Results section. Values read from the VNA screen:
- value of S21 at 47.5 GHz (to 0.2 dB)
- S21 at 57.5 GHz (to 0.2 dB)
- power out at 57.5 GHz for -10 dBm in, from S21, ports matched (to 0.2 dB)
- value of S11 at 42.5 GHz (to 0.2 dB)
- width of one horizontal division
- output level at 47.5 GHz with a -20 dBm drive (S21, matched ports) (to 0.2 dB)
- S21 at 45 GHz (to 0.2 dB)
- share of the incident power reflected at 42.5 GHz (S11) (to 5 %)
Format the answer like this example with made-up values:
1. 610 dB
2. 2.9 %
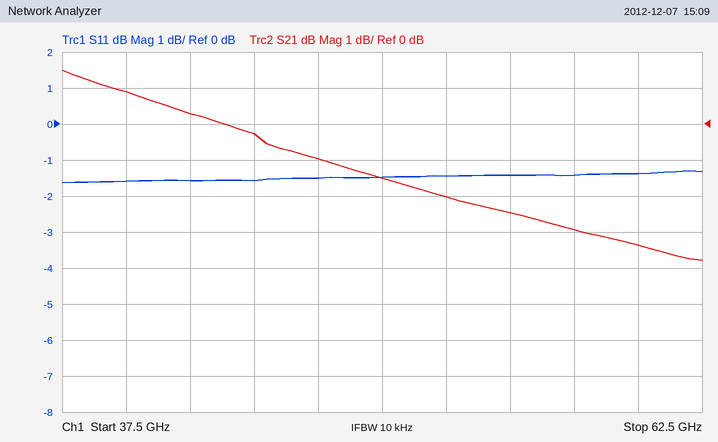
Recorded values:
1. -1.0 dB
2. -3.0 dB
3. -13.0 dBm
4. -1.6 dB
5. 2.5 GHz
6. -21.0 dBm
7. -0.2 dB
8. 70 %
